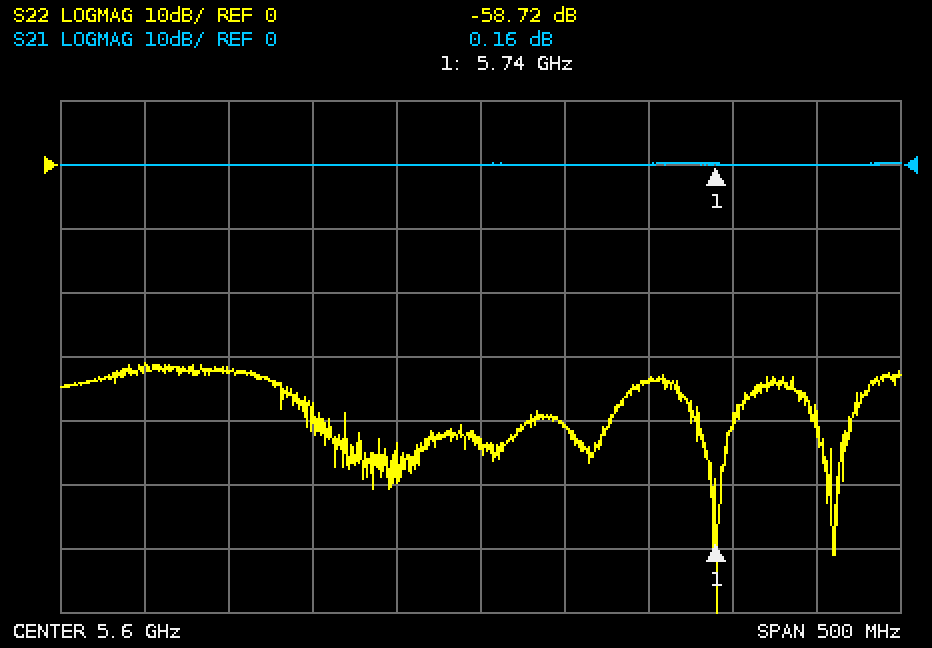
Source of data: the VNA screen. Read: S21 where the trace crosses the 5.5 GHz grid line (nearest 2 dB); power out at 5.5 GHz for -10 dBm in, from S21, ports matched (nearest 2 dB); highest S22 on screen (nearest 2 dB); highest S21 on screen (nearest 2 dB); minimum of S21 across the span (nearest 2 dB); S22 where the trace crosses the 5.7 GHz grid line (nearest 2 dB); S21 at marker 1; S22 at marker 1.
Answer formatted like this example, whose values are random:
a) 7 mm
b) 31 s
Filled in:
a) 0 dB
b) -10 dBm
c) -30 dB
d) 0 dB
e) 0 dB
f) -34 dB
g) 0.16 dB
h) -58.72 dB
